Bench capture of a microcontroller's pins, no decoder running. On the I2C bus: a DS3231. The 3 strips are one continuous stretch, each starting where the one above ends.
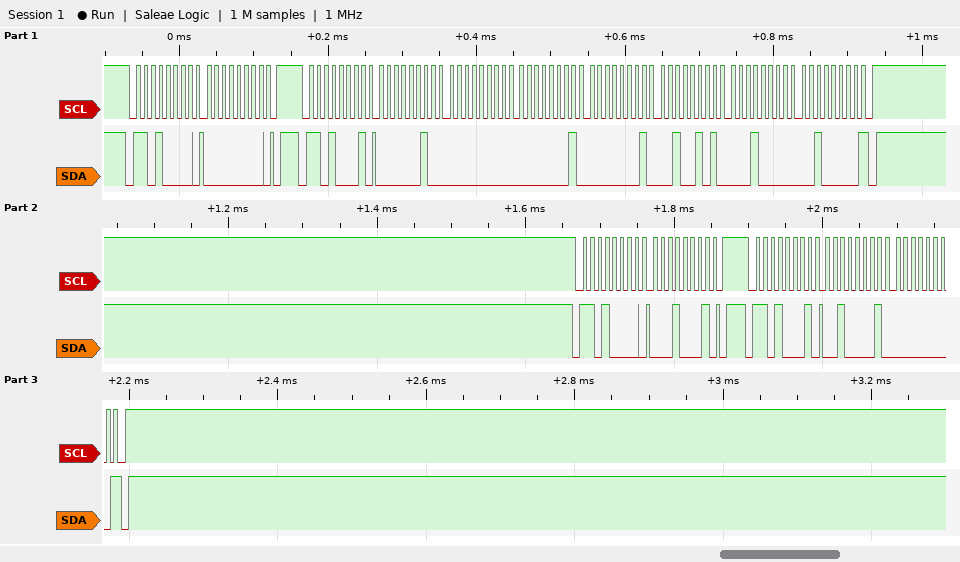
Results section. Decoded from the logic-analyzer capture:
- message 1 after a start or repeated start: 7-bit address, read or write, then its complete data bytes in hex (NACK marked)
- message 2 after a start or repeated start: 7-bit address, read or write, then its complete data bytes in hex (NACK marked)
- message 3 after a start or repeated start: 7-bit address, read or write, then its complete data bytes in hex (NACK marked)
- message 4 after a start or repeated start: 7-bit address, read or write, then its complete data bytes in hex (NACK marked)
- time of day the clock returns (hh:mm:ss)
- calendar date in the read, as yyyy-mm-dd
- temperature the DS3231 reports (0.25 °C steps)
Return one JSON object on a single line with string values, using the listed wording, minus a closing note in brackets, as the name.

{"message 1 after a start or repeated start: 7-bit address, read or write, then its complete data bytes in hex": "0x68 write: 00", "message 2 after a start or repeated start: 7-bit address, read or write, then its complete data bytes in hex": "0x68 read: 02 00 01 01 25 10 20 NACK", "message 3 after a start or repeated start: 7-bit address, read or write, then its complete data bytes in hex": "0x68 write: 11", "message 4 after a start or repeated start: 7-bit address, read or write, then its complete data bytes in hex": "0x68 read: 21 00 NACK", "time of day the clock returns": "01:00:02", "calendar date in the read, as yyyy-mm-dd": "2020-10-25", "temperature the DS3231 reports": "33.00 °C"}
